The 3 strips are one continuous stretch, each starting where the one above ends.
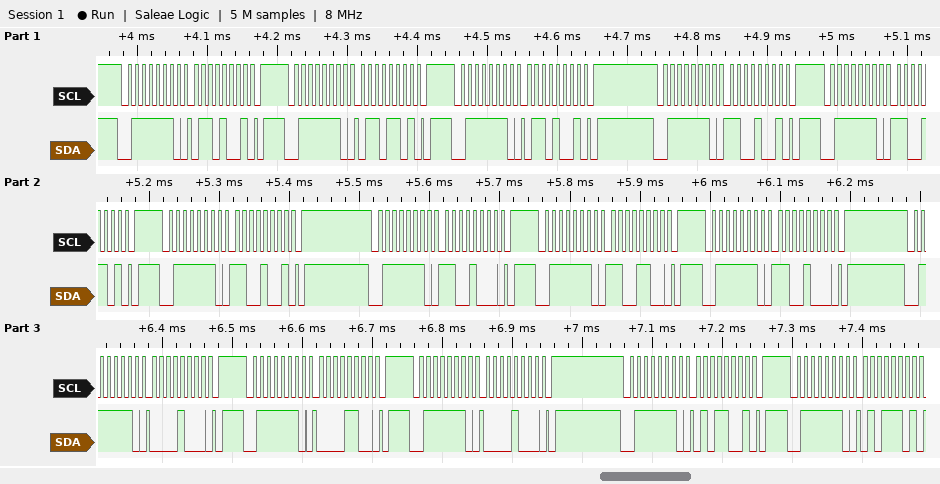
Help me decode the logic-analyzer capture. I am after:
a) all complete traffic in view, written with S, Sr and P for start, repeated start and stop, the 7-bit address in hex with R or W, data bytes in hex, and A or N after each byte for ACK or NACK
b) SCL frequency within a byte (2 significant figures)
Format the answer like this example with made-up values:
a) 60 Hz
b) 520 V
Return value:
a) S 3FW A 69 A P S 3FW A 6D A P S 3FW A 69 A P S 3FW A C9 A P S 3FW A CD A P S 3FW A C9 A P S 3FW A C8 A P S 3FW A CC A P S 3FW A C8 A P S 3FW A 08 A P S 3FW A 0C A P S 3FW A 08 A P S 3FW A 59 A P S 3FW A 5D A
b) 100 kHz
